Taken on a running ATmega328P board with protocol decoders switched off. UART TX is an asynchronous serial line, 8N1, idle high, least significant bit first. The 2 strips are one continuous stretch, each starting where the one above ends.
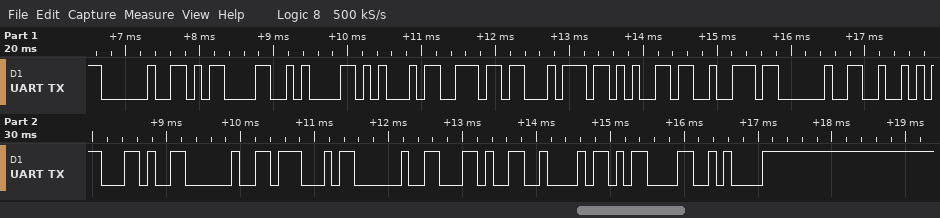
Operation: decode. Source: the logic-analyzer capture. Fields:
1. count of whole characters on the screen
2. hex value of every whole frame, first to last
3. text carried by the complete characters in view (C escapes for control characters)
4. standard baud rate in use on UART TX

18
20 0D 0A 45 6E 74 65 72 20 52 2C 20 47 20 2C 42 0D 0A
" \r\nEnter R, G ,B\r\n"
9600 baud
